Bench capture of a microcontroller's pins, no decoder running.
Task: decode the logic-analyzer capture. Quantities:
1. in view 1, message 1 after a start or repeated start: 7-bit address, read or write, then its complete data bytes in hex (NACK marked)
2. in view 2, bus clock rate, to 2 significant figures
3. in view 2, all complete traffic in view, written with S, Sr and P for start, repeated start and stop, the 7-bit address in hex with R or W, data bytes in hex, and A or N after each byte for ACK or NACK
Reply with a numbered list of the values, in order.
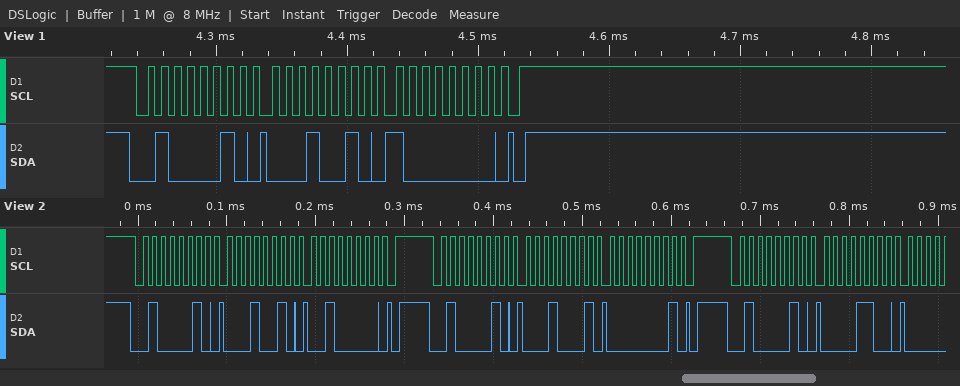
1. 0x21 write: 12 80
2. 100 kHz
3. S 21W A 12 A 20 A P S 21W A 11 A 01 A P S 21W A 0C A
